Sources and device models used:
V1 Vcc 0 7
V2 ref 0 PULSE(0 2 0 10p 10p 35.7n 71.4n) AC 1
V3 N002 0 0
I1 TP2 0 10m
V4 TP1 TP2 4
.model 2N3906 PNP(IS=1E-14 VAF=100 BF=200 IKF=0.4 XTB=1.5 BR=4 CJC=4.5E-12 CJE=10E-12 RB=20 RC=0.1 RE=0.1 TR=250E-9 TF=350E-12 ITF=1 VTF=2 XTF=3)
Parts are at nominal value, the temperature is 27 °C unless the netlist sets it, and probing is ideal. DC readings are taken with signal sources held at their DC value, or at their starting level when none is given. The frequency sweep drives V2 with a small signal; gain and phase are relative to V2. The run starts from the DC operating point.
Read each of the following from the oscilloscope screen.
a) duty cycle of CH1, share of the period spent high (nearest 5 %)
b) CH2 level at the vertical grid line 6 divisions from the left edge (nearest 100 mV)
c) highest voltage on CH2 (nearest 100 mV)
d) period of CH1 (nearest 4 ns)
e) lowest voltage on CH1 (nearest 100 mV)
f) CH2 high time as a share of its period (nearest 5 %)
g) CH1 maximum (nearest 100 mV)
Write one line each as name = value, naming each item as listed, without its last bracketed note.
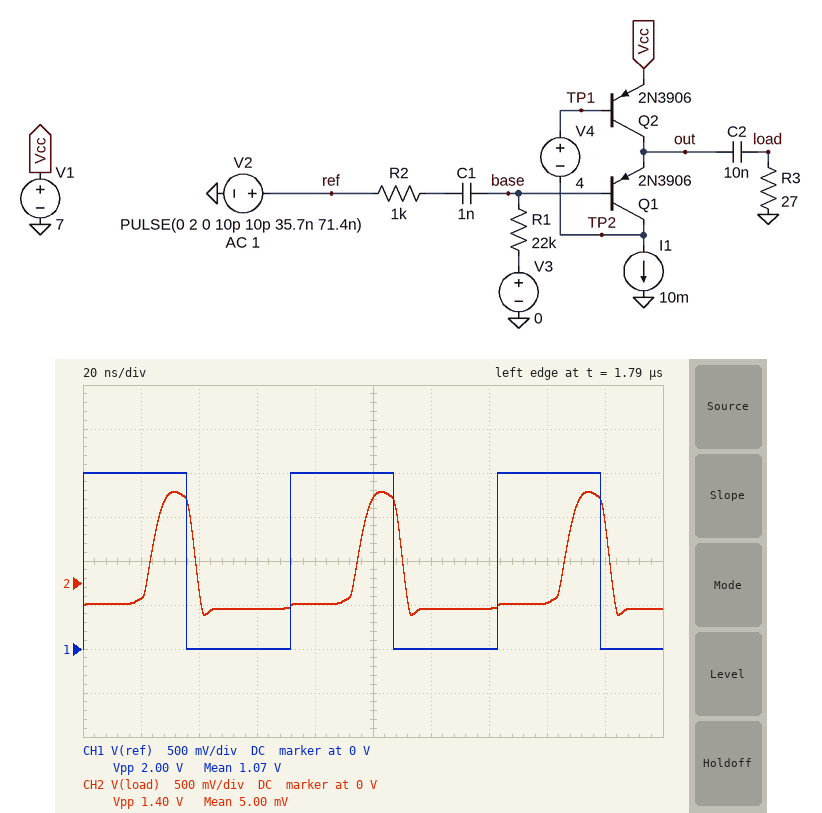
duty cycle of CH1, share of the period spent high = 50 %
CH2 level at the vertical grid line 6 divisions from the left edge = -300 mV
highest voltage on CH2 = 1.0 V
period of CH1 = 72 ns
lowest voltage on CH1 = 0 V
CH2 high time as a share of its period = 20 %
CH1 maximum = 2.0 V
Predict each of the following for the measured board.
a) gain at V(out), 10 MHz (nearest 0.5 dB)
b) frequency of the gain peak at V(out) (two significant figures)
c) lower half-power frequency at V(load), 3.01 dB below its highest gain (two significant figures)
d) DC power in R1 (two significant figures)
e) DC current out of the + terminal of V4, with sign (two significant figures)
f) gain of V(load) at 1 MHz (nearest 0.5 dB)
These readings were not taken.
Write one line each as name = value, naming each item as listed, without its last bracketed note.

gain at V(out), 10 MHz = -37.0 dB
frequency of the gain peak at V(out) = 160 kHz
lower half-power frequency at V(load), 3.01 dB below its highest gain = 210 kHz
DC power in R1 = 130 µW
DC current out of the + terminal of V4, with sign = -49 µA
gain of V(load) at 1 MHz = -18.5 dB
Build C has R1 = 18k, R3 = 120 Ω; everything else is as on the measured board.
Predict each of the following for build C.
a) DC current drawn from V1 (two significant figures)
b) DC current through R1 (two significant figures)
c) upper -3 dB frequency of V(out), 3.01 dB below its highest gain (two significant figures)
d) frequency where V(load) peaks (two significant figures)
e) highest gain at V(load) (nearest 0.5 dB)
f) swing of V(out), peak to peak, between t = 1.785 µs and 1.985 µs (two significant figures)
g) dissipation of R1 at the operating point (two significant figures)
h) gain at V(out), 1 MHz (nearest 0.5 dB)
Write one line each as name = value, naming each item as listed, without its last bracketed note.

DC current drawn from V1 = 10 mA
DC current through R1 = 93 µA
upper -3 dB frequency of V(out), 3.01 dB below its highest gain = 470 kHz
frequency where V(load) peaks = 240 kHz
highest gain at V(load) = -14.5 dB
swing of V(out), peak to peak, between t = 1.785 µs and 1.985 µs = 1.6 V
dissipation of R1 at the operating point = 160 µW
gain at V(out), 1 MHz = -21.0 dB
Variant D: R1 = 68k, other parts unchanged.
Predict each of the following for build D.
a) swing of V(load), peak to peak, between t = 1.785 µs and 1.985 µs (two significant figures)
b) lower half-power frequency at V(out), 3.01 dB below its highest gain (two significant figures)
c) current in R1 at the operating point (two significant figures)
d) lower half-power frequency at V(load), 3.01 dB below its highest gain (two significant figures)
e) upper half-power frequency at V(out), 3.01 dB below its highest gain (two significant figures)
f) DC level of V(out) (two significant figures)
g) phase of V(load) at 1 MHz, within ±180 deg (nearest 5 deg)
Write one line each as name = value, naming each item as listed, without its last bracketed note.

swing of V(load), peak to peak, between t = 1.785 µs and 1.985 µs = 1.6 V
lower half-power frequency at V(out), 3.01 dB below its highest gain = 2.5 kHz
current in R1 at the operating point = 50 µA
lower half-power frequency at V(load), 3.01 dB below its highest gain = 610 kHz
upper half-power frequency at V(out), 3.01 dB below its highest gain = 52 MHz
DC level of V(out) = 4.1 V
phase of V(load) at 1 MHz, within ±180 deg = 30 deg
